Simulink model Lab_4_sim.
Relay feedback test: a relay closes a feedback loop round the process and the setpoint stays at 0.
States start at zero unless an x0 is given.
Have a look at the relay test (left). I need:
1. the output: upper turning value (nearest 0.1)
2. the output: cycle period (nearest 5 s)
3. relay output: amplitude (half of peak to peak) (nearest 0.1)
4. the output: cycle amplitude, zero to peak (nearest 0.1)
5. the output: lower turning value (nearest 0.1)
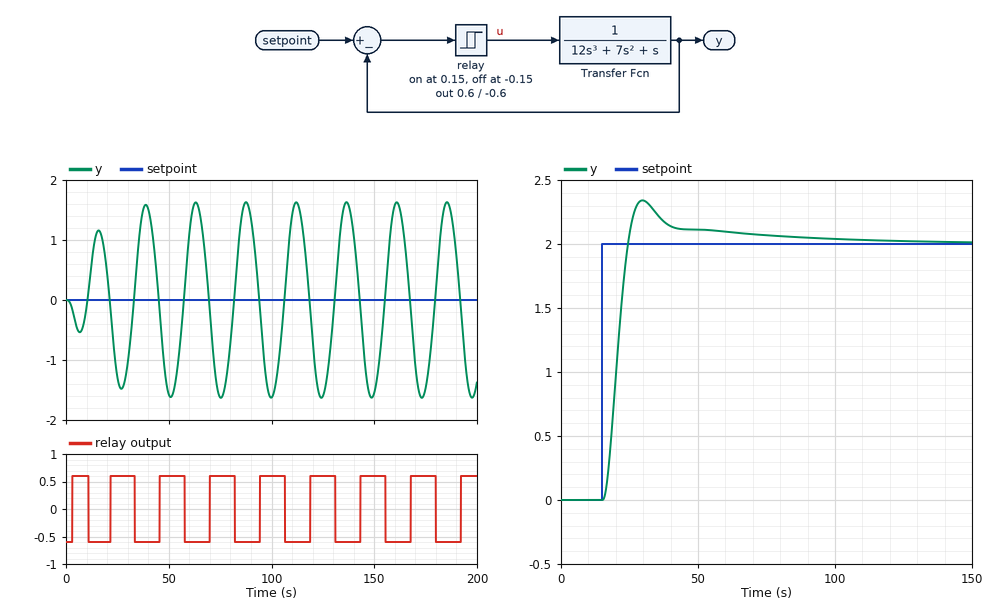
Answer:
1.6
25 s
0.6
1.6
-1.6
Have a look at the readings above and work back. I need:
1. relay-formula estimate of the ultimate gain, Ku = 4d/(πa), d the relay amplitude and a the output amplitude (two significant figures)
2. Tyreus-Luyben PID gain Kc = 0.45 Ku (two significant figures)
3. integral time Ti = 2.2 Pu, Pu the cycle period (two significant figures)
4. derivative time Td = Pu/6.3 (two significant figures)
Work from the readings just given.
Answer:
0.48
0.22
55 s
4.0 s
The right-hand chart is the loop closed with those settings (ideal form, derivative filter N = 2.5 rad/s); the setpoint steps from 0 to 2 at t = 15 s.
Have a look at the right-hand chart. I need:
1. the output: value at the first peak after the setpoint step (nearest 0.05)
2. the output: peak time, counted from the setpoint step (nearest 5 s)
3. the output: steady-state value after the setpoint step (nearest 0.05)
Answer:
2.35
15 s
2.00
